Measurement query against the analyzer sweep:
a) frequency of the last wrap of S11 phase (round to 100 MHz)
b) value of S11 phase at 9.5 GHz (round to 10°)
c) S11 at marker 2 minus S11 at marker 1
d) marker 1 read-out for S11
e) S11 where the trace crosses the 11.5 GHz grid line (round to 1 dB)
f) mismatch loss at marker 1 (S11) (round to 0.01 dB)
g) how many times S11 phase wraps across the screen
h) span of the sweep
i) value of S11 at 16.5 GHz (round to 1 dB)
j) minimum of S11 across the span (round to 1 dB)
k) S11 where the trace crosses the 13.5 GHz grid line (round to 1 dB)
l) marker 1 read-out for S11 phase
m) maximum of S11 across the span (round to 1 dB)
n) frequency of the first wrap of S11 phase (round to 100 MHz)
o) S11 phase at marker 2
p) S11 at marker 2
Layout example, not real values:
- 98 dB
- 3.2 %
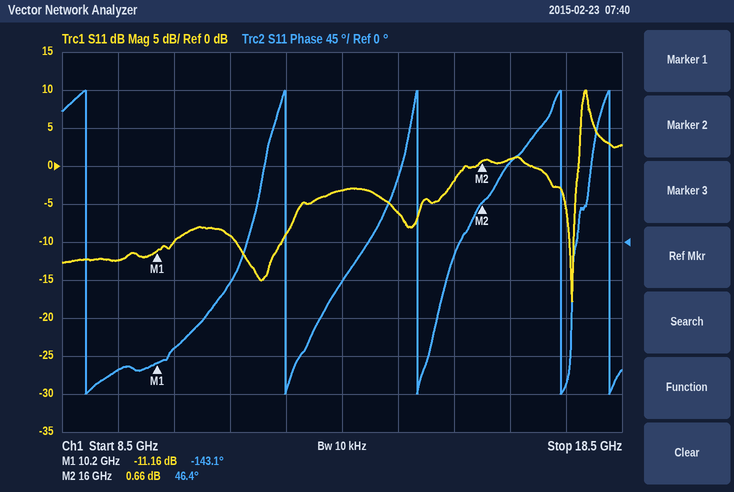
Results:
- 18.3 GHz
- -150°
- 11.82 dB
- -11.16 dB
- -9 dB
- 0.35 dB
- 5
- 10 GHz
- 1 dB
- -18 dB
- -3 dB
- -143.1°
- 10 dB
- 8.9 GHz
- 46.4°
- 0.66 dB
